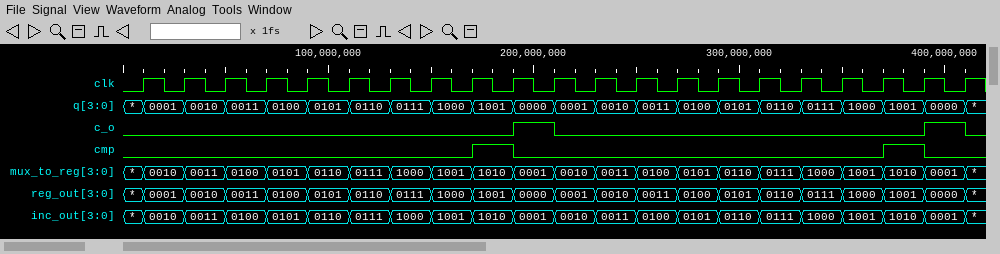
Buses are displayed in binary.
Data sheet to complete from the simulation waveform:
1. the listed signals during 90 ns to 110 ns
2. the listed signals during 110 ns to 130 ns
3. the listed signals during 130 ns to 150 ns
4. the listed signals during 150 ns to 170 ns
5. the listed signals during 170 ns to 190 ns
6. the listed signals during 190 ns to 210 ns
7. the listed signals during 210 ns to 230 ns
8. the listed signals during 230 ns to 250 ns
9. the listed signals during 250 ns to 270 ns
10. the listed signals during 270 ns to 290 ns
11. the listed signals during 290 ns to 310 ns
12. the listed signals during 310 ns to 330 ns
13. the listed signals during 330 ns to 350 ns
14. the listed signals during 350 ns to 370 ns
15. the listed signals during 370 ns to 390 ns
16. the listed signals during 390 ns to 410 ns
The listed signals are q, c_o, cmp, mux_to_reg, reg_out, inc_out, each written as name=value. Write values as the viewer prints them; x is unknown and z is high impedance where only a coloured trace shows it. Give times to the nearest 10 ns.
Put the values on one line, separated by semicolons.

q=0101, c_o=0, cmp=0, mux_to_reg=0110, reg_out=0101, inc_out=0110; q=0110, c_o=0, cmp=0, mux_to_reg=0111, reg_out=0110, inc_out=0111; q=0111, c_o=0, cmp=0, mux_to_reg=1000, reg_out=0111, inc_out=1000; q=1000, c_o=0, cmp=0, mux_to_reg=1001, reg_out=1000, inc_out=1001; q=1001, c_o=0, cmp=1, mux_to_reg=1010, reg_out=1001, inc_out=1010; q=0000, c_o=1, cmp=0, mux_to_reg=0001, reg_out=0000, inc_out=0001; q=0001, c_o=0, cmp=0, mux_to_reg=0010, reg_out=0001, inc_out=0010; q=0010, c_o=0, cmp=0, mux_to_reg=0011, reg_out=0010, inc_out=0011; q=0011, c_o=0, cmp=0, mux_to_reg=0100, reg_out=0011, inc_out=0100; q=0100, c_o=0, cmp=0, mux_to_reg=0101, reg_out=0100, inc_out=0101; q=0101, c_o=0, cmp=0, mux_to_reg=0110, reg_out=0101, inc_out=0110; q=0110, c_o=0, cmp=0, mux_to_reg=0111, reg_out=0110, inc_out=0111; q=0111, c_o=0, cmp=0, mux_to_reg=1000, reg_out=0111, inc_out=1000; q=1000, c_o=0, cmp=0, mux_to_reg=1001, reg_out=1000, inc_out=1001; q=1001, c_o=0, cmp=1, mux_to_reg=1010, reg_out=1001, inc_out=1010; q=0000, c_o=1, cmp=0, mux_to_reg=0001, reg_out=0000, inc_out=0001
